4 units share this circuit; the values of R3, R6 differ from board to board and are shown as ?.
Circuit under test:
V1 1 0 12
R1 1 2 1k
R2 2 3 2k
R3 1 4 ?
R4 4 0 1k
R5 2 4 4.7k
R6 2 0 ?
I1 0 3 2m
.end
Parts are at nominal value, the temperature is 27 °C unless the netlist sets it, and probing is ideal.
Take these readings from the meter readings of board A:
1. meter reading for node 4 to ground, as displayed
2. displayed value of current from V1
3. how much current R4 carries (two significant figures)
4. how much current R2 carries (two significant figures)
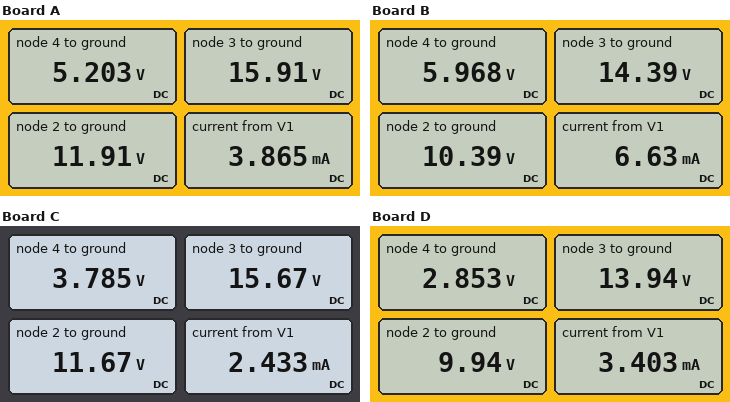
5.203 V
3.865 mA
5.2 mA
2.0 mA
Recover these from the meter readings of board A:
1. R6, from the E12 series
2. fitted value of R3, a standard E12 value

18 kΩ
1.8 kΩ
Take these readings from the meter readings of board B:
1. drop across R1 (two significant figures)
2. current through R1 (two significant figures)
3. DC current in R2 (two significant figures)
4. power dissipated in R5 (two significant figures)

1.6 V
1.6 mA
2.0 mA
4.2 mW
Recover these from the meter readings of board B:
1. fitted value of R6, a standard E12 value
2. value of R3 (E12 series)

3.9 kΩ
1.2 kΩ
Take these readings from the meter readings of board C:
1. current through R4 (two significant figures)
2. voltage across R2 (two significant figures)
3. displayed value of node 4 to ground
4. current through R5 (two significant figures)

3.8 mA
4.0 V
3.785 V
1.7 mA
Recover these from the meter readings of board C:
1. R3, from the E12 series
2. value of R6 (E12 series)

3.9 kΩ
18 kΩ
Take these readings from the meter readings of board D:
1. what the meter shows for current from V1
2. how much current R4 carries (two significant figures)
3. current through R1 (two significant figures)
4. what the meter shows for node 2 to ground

3.403 mA
2.9 mA
2.1 mA
9.94 V
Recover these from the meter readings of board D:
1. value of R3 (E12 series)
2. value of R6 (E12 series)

6.8 kΩ
3.9 kΩ
